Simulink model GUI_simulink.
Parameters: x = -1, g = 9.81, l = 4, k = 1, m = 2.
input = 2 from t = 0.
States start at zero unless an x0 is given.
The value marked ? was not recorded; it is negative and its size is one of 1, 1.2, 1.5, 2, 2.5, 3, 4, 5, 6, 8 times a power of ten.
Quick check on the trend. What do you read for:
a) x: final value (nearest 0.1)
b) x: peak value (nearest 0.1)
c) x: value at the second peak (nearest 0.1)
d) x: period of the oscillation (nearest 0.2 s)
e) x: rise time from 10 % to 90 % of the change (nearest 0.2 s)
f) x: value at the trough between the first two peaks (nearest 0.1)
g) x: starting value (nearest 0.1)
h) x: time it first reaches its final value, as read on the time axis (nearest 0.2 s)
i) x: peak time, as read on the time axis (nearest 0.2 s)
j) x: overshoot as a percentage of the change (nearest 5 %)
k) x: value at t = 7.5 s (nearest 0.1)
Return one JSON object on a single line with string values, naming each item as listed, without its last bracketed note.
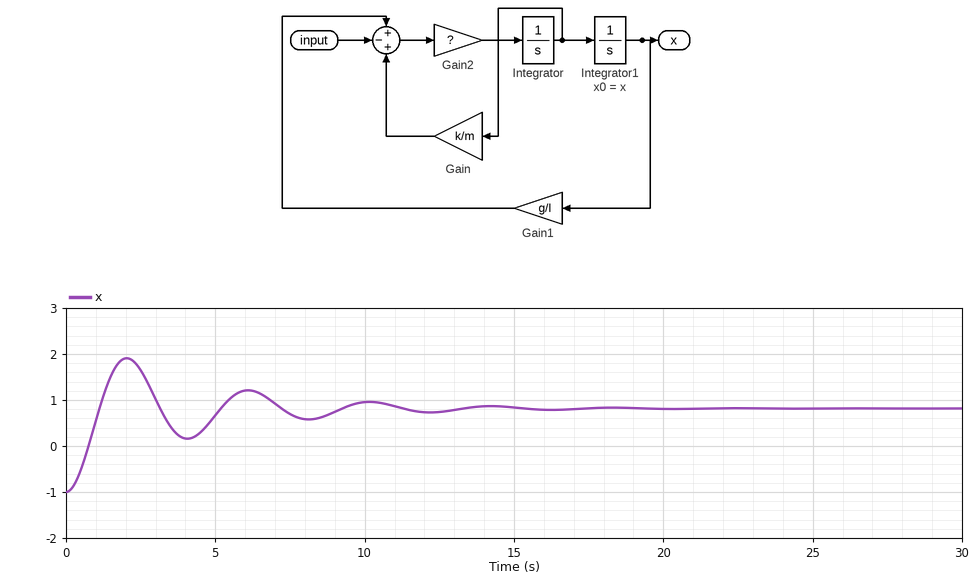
{"x: final value": "0.8", "x: peak value": "1.9", "x: value at the second peak": "1.2", "x: period of the oscillation": "4.0 s", "x: rise time from 10 % to 90 % of the change": "0.8 s", "x: value at the trough between the first two peaks": "0.2", "x: starting value": "-1.0", "x: time it first reaches its final value, as read on the time axis": "1.2 s", "x: peak time, as read on the time axis": "2.0 s", "x: overshoot as a percentage of the change": "60 %", "x: value at t = 7.5 s": "0.7"}
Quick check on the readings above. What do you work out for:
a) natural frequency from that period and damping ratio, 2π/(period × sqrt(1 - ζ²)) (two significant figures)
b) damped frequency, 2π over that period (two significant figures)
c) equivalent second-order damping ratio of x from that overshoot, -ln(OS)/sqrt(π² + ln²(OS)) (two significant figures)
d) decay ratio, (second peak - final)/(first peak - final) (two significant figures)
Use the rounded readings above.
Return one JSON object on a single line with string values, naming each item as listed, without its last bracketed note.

{"natural frequency from that period and damping ratio, 2π/(period × sqrt(1 - ζ²))": "1.6 rad/s", "damped frequency, 2π over that period": "1.6 rad/s", "equivalent second-order damping ratio of x from that overshoot, -ln(OS)/sqrt(π² + ln²(OS))": "0.16", "decay ratio, (second peak - final)/(first peak - final)": "0.36"}
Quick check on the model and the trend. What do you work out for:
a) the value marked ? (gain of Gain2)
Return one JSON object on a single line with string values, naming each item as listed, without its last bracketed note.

{"the value marked ?": "-1"}
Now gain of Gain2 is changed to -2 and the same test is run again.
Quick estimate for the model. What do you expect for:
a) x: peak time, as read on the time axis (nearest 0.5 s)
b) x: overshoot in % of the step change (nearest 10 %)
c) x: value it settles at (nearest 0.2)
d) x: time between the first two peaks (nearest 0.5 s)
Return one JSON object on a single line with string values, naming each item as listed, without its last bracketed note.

{"x: peak time, as read on the time axis": "1.5 s", "x: overshoot in % of the step change": "50 %", "x: value it settles at": "0.8", "x: time between the first two peaks": "3.0 s"}
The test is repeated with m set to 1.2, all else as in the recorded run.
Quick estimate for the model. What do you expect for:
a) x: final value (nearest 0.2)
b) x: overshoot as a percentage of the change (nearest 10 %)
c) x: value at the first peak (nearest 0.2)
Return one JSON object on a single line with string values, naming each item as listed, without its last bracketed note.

{"x: final value": "0.8", "x: overshoot as a percentage of the change": "40 %", "x: value at the first peak": "1.6"}
